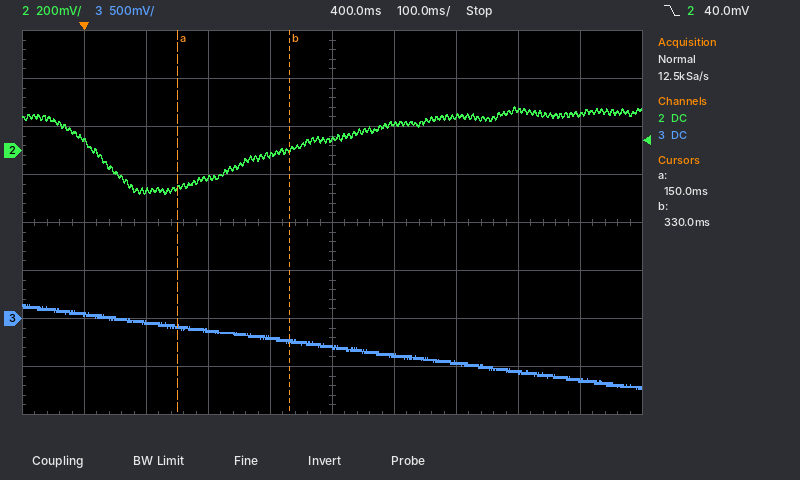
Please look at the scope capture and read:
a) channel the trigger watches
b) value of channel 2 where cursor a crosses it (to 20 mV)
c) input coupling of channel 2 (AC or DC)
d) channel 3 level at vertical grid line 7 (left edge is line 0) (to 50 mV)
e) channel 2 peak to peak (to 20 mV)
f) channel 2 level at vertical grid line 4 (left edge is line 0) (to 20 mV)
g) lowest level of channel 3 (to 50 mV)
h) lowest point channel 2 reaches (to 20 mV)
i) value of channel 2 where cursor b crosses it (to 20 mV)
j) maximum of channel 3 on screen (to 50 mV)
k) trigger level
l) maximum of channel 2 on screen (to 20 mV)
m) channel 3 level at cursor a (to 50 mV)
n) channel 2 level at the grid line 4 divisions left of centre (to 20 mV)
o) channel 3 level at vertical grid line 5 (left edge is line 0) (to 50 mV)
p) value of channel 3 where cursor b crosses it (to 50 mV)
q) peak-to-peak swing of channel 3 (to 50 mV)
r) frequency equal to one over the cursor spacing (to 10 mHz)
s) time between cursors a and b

channel 2
-160 mV
DC
-450 mV
360 mV
-20 mV
-750 mV
-180 mV
0 mV
150 mV
40.0 mV
180 mV
-100 mV
40 mV
-300 mV
-250 mV
900 mV
5.56 Hz
180 ms
